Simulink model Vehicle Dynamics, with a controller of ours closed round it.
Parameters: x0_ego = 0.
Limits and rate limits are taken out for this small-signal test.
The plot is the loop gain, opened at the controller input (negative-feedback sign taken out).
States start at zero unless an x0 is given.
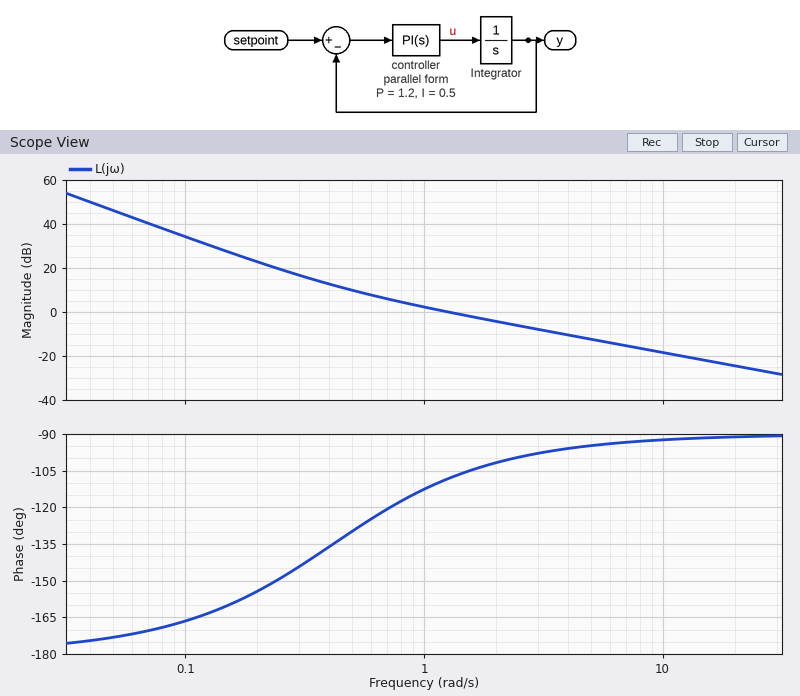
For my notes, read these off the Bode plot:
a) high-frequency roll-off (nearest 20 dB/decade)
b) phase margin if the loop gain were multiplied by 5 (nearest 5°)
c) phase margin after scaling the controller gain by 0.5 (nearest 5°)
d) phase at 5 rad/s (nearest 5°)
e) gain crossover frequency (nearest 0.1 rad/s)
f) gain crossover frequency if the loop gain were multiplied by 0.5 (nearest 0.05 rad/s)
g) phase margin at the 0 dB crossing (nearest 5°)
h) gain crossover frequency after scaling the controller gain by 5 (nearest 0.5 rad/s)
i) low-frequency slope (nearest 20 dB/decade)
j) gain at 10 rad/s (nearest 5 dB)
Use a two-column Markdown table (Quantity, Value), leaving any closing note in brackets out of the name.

| Quantity | Value |
|---|---|
| high-frequency roll-off | -20 dB/decade |
| phase margin if the loop gain were multiplied by 5 | 85° |
| phase margin after scaling the controller gain by 0.5 | 60° |
| phase at 5 rad/s | -95° |
| gain crossover frequency | 1.3 rad/s |
| gain crossover frequency if the loop gain were multiplied by 0.5 | 0.70 rad/s |
| phase margin at the 0 dB crossing | 70° |
| gain crossover frequency after scaling the controller gain by 5 | 6.0 rad/s |
| low-frequency slope | -40 dB/decade |
| gain at 10 rad/s | -20 dB |
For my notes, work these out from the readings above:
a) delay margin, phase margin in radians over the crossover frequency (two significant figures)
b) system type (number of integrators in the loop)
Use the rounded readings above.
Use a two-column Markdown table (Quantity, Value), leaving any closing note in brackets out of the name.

| Quantity | Value |
|---|---|
| delay margin, phase margin in radians over the crossover frequency | 0.94 s |
| system type | 2 |
